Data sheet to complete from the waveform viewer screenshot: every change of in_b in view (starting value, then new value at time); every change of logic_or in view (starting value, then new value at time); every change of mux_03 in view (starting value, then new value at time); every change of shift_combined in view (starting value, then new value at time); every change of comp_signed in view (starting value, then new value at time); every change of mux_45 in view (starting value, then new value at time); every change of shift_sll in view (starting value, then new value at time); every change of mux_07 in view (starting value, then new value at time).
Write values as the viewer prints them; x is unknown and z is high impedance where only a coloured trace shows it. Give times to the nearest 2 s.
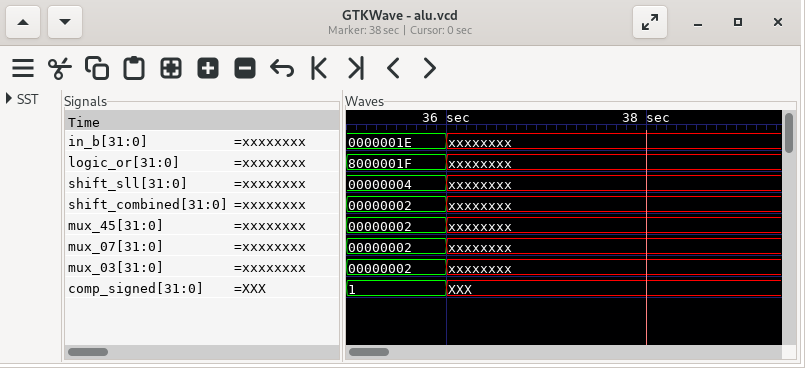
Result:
0000001E, xxxxxxxx at 36 s
8000001F, xxxxxxxx at 36 s
00000002, xxxxxxxx at 36 s
00000002, xxxxxxxx at 36 s
1, XXX at 36 s
00000002, xxxxxxxx at 36 s
00000004, xxxxxxxx at 36 s
00000002, xxxxxxxx at 36 s
